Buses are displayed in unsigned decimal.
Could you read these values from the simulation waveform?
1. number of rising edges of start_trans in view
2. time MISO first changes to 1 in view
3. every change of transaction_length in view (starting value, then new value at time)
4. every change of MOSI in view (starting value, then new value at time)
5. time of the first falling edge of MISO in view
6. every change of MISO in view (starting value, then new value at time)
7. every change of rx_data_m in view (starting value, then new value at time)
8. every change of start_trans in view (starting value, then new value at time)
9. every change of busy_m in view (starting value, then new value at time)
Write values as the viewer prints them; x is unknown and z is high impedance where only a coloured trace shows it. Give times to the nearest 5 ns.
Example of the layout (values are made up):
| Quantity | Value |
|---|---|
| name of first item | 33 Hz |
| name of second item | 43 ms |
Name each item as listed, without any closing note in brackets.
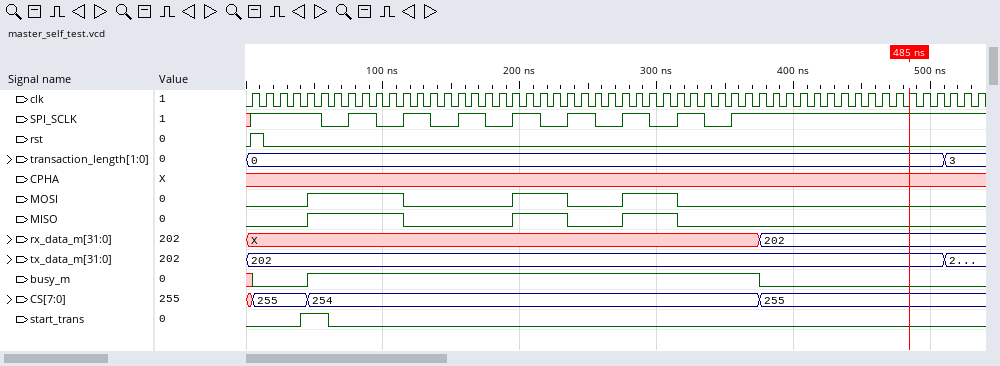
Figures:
| Quantity | Value |
|---|---|
| number of rising edges of start_trans in view | 1 |
| time MISO first changes to 1 in view | 45 ns |
| every change of transaction_length in view | 0, 3 at 510 ns |
| every change of MOSI in view | 0, 1 at 45 ns, 0 at 115 ns, 1 at 195 ns, 0 at 235 ns, 1 at 275 ns, 0 at 315 ns |
| time of the first falling edge of MISO in view | 115 ns |
| every change of MISO in view | 0, 1 at 45 ns, 0 at 115 ns, 1 at 195 ns, 0 at 235 ns, 1 at 275 ns, 0 at 315 ns |
| every change of rx_data_m in view | X, 202 at 375 ns |
| every change of start_trans in view | 0, 1 at 40 ns, 0 at 60 ns |
| every change of busy_m in view | x, 0 at 5 ns, 1 at 45 ns, 0 at 375 ns |
